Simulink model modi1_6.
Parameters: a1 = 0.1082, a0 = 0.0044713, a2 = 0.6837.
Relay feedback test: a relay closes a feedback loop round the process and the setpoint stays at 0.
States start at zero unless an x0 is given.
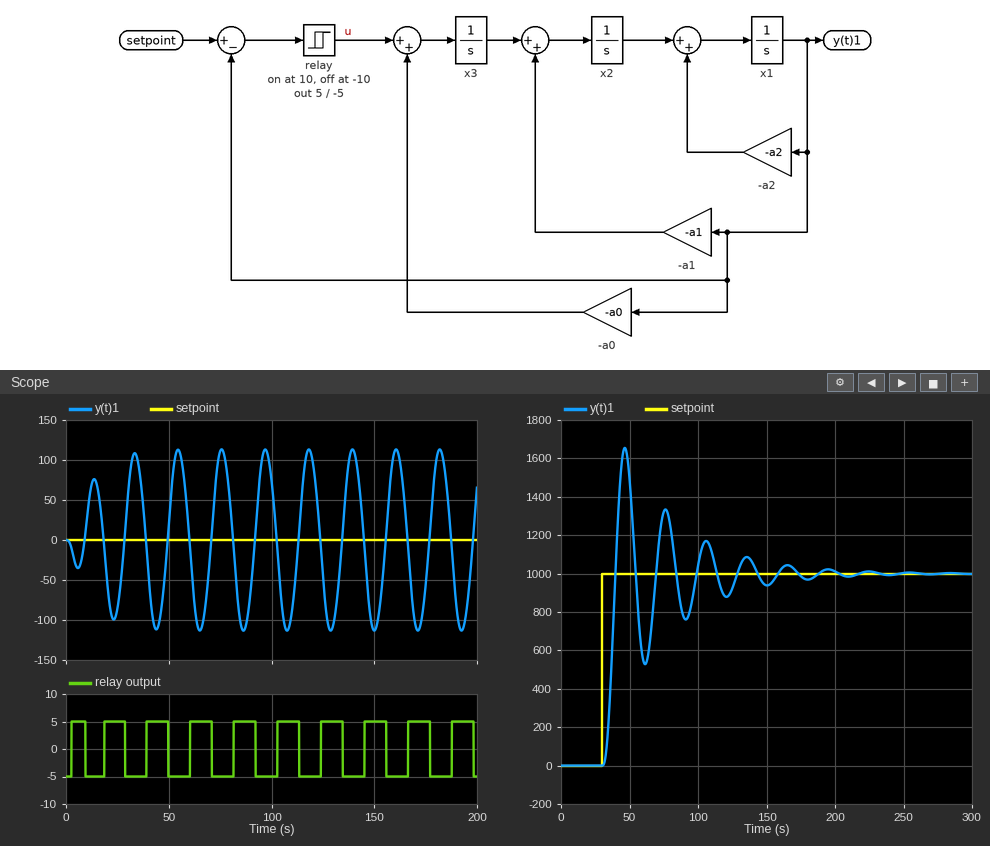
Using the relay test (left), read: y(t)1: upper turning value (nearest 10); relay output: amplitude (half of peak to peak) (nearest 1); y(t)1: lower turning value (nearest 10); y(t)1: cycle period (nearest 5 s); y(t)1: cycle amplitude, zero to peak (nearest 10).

110
5
-110
20 s
110
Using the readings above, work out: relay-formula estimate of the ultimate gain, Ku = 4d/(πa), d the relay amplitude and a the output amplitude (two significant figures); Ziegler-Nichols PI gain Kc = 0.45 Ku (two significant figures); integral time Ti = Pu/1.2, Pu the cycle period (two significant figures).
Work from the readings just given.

0.058
0.026
17 s
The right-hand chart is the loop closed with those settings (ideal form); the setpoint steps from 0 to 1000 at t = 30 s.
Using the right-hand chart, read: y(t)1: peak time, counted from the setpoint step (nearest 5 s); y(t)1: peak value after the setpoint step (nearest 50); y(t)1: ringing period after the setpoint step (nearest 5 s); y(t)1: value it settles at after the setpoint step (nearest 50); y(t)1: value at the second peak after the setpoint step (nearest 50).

15 s
1650
30 s
1000
1350
